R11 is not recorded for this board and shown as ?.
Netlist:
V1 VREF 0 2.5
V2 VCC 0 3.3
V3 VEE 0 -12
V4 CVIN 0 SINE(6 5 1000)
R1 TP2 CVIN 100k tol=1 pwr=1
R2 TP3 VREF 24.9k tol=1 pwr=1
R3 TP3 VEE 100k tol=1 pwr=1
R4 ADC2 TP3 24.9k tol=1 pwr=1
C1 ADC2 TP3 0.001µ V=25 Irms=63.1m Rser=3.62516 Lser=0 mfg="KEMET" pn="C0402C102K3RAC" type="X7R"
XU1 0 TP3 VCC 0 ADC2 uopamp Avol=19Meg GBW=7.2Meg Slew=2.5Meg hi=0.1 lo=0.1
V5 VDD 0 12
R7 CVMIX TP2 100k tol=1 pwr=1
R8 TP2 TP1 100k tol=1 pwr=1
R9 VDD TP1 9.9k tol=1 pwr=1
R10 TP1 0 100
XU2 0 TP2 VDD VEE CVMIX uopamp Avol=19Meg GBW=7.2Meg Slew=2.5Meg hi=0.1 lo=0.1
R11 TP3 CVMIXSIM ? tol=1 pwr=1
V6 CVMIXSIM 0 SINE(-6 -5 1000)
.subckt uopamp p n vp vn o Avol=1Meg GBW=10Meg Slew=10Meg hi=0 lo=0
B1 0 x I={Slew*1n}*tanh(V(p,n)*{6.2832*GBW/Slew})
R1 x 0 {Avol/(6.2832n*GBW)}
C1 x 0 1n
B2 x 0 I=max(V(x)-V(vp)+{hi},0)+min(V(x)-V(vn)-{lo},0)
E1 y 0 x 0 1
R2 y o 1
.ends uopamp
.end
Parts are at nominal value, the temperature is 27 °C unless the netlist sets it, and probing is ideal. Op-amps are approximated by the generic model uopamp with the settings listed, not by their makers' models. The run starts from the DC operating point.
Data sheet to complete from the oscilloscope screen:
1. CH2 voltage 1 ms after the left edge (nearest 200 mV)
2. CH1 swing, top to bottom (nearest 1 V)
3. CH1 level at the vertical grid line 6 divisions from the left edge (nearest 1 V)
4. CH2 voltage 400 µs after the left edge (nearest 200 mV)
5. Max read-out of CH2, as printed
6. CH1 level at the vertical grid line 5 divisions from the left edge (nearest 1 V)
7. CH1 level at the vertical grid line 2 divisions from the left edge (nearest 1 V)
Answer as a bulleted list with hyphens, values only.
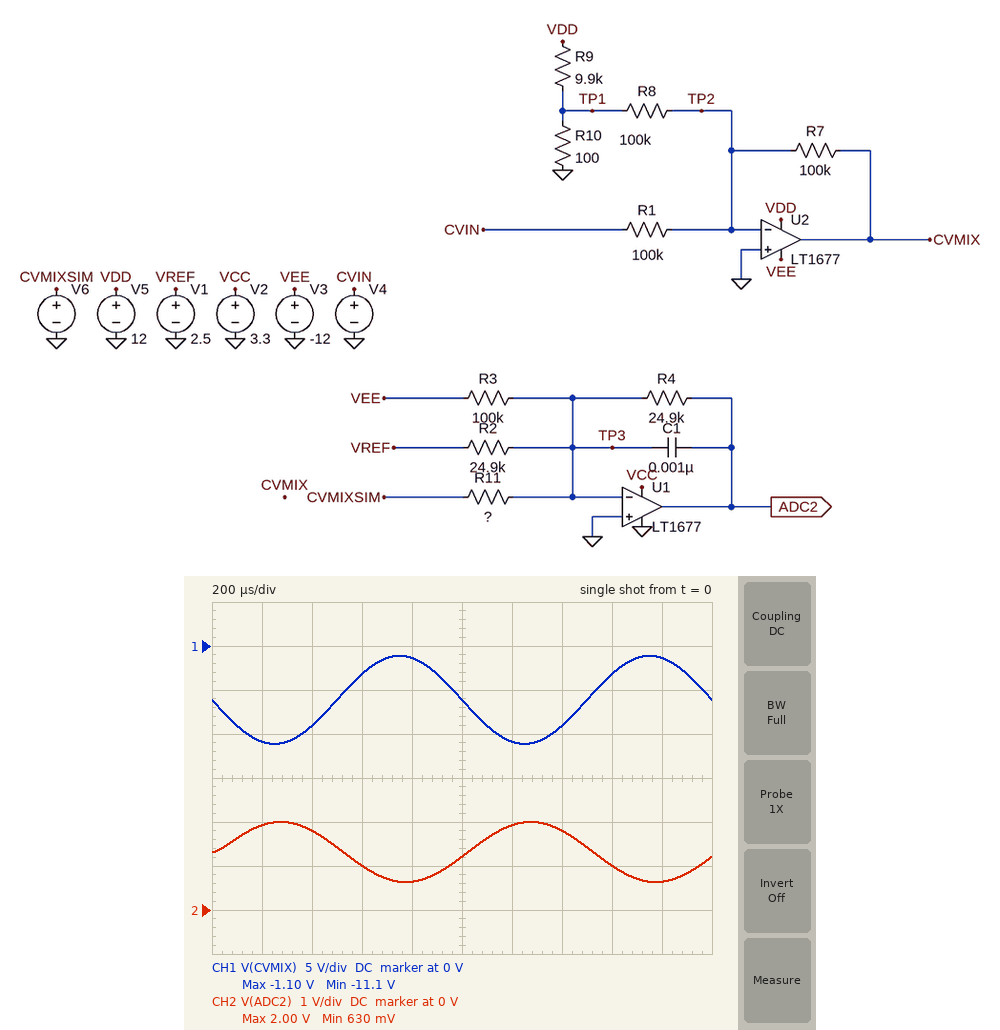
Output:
- 1.2 V
- 10 V
- -11 V
- 1.8 V
- 2.00 V
- -6 V
- -9 V
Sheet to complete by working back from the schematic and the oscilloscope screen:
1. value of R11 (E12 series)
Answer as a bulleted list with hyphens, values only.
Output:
- 180 kΩ
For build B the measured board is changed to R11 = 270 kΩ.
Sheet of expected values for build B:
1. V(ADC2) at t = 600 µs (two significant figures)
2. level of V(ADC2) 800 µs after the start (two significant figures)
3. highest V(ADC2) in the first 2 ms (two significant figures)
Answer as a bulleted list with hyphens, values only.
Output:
- 830 mV
- 590 mV
- 1.5 V
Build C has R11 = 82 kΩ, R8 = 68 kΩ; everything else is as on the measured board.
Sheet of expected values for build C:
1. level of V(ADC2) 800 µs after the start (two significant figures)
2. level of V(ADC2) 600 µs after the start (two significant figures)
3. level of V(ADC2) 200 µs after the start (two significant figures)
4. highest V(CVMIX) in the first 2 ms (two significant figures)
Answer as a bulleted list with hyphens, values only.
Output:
- 830 mV
- 1.6 V
- 3.2 V
- -1.2 V
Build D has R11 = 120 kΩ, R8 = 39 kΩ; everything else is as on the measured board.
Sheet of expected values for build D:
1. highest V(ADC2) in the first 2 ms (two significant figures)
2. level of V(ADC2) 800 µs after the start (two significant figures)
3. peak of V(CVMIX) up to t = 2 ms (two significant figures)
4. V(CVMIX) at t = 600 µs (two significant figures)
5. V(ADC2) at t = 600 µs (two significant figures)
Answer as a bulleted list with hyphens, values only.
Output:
- 2.8 V
- 720 mV
- -1.3 V
- -3.4 V
- 1.3 V
